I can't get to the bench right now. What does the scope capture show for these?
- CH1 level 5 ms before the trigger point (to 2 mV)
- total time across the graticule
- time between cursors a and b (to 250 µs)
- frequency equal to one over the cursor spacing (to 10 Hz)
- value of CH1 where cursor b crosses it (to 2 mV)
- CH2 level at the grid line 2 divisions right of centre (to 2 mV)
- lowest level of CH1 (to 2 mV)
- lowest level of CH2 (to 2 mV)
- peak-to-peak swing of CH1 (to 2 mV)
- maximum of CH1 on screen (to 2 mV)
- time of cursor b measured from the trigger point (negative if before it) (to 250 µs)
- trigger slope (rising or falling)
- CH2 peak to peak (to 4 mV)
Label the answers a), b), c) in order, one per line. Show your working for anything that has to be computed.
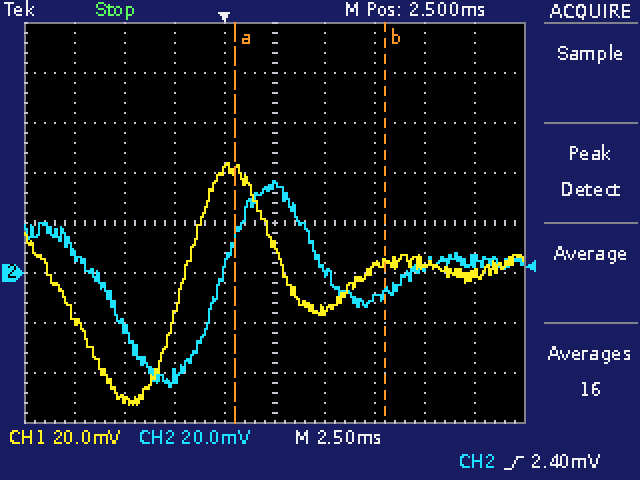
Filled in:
a) -50 mV
b) 25 ms
c) 7.50 ms
d) 1 / 7.50 ms ≈ 130 Hz
e) 4 mV
f) -10 mV
g) -52 mV
h) -46 mV
i) 44 mV − (-52 mV) = 96 mV
j) 44 mV
k) +8.00 ms
l) rising
m) 84 mV
